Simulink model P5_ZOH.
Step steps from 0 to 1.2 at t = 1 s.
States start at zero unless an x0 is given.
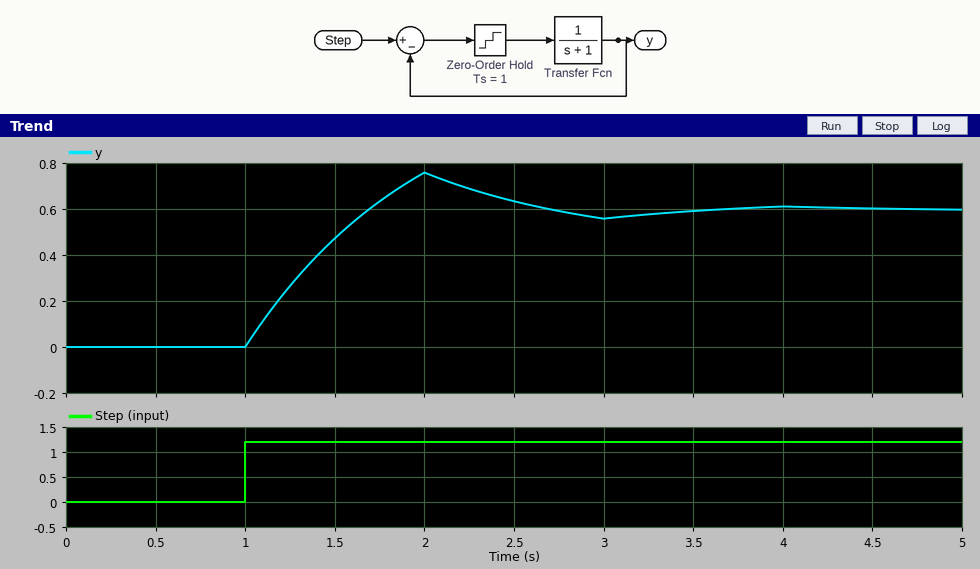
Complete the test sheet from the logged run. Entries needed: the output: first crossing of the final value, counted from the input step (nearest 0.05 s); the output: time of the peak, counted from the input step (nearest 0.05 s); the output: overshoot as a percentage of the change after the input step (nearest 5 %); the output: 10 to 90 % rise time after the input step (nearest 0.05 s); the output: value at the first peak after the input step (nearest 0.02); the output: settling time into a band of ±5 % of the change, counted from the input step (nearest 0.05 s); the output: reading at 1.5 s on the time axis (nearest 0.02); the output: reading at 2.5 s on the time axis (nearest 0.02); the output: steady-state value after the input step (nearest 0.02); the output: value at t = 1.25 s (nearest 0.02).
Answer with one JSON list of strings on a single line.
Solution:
["0.70 s", "1.00 s", "25 %", "0.55 s", "0.76", "2.15 s", "0.48", "0.64", "0.60", "0.26"]
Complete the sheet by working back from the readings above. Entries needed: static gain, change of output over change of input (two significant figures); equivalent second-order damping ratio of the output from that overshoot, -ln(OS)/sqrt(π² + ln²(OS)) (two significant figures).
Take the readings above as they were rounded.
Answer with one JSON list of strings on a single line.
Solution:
["0.50", "0.40"]
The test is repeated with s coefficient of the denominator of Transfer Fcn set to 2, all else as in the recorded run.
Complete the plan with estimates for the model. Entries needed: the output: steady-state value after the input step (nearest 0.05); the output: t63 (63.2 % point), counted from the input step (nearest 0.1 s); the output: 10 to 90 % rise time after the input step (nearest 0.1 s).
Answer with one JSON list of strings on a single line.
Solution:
["0.60", "0.8 s", "1.5 s"]
